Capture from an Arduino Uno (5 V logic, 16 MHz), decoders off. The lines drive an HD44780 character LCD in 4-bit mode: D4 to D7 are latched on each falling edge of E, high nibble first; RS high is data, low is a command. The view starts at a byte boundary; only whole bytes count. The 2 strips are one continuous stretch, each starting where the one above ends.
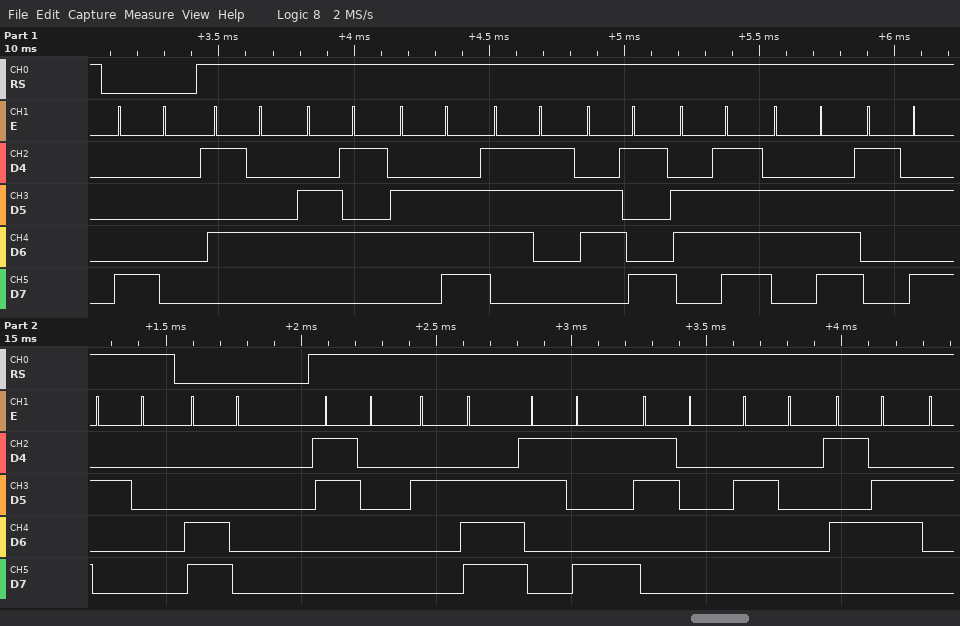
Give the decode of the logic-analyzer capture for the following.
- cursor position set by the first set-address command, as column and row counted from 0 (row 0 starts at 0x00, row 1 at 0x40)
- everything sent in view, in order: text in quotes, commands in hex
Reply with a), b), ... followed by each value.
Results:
a) column 0, row 0
b) 0x80 "Tension: " 0xC0 "0.90 V"
